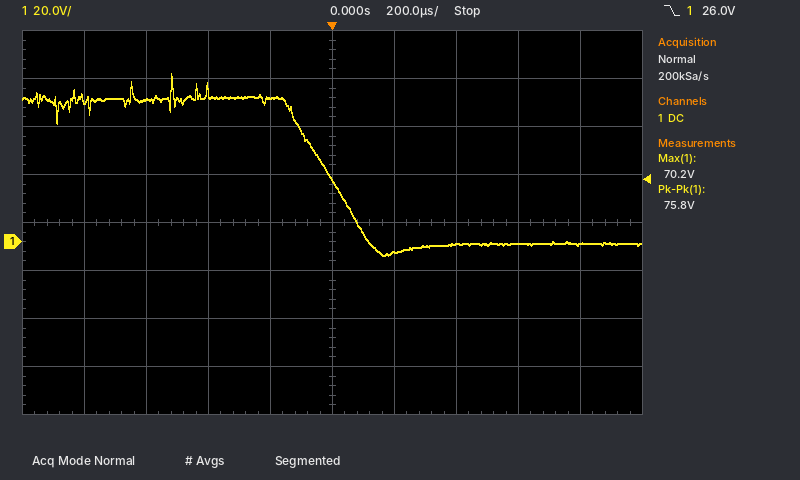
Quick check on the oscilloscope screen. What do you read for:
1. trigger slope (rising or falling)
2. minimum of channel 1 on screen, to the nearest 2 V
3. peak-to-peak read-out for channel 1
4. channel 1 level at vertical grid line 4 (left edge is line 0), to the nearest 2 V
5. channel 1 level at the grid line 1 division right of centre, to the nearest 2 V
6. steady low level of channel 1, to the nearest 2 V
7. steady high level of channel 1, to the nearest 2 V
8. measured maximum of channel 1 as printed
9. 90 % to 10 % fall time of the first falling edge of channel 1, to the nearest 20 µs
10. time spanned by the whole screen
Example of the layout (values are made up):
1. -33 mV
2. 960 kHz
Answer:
1. falling
2. -6 V
3. 75.8 V
4. 60 V
5. -4 V
6. 0 V
7. 60 V
8. 70.2 V
9. 220 µs
10. 2 ms
